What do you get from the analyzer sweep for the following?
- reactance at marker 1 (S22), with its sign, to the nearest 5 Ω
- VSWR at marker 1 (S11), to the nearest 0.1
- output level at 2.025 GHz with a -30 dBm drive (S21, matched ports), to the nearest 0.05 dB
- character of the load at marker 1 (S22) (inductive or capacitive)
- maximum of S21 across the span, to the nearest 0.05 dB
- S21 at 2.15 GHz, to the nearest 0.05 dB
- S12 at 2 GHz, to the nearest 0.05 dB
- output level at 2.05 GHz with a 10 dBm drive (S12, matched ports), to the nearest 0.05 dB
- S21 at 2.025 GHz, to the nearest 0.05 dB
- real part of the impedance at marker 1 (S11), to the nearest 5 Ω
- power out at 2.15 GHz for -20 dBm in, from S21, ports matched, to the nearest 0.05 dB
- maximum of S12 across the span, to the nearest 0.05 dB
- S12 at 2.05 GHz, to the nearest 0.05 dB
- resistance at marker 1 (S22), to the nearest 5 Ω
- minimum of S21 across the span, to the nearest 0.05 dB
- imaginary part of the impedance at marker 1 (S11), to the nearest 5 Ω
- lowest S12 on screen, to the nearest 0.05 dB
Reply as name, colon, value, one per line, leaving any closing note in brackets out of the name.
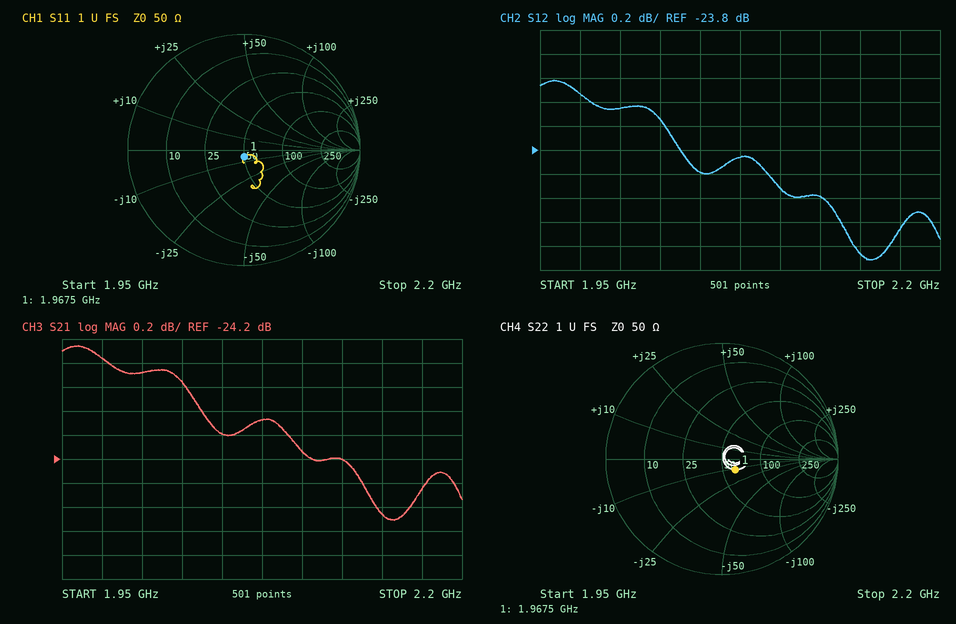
reactance at marker 1 (S22), with its sign, to the nearest 5 Ω: -10 Ω
VSWR at marker 1 (S11), to the nearest 0.1: 1.1
output level at 2.025 GHz with a -30 dBm drive (S21, matched ports), to the nearest 0.05 dB: -53.55 dBm
character of the load at marker 1 (S22): capacitive
maximum of S21 across the span, to the nearest 0.05 dB: -23.25 dB
S21 at 2.15 GHz, to the nearest 0.05 dB: -24.65 dB
S12 at 2 GHz, to the nearest 0.05 dB: -23.45 dB
output level at 2.05 GHz with a 10 dBm drive (S12, matched ports), to the nearest 0.05 dB: -14.00 dBm
S21 at 2.025 GHz, to the nearest 0.05 dB: -23.55 dB
real part of the impedance at marker 1 (S11), to the nearest 5 Ω: 50 Ω
power out at 2.15 GHz for -20 dBm in, from S21, ports matched, to the nearest 0.05 dB: -44.65 dBm
maximum of S12 across the span, to the nearest 0.05 dB: -23.20 dB
S12 at 2.05 GHz, to the nearest 0.05 dB: -24.00 dB
resistance at marker 1 (S22), to the nearest 5 Ω: 60 Ω
minimum of S21 across the span, to the nearest 0.05 dB: -24.70 dB
imaginary part of the impedance at marker 1 (S11), to the nearest 5 Ω: -5 Ω
lowest S12 on screen, to the nearest 0.05 dB: -24.70 dB
